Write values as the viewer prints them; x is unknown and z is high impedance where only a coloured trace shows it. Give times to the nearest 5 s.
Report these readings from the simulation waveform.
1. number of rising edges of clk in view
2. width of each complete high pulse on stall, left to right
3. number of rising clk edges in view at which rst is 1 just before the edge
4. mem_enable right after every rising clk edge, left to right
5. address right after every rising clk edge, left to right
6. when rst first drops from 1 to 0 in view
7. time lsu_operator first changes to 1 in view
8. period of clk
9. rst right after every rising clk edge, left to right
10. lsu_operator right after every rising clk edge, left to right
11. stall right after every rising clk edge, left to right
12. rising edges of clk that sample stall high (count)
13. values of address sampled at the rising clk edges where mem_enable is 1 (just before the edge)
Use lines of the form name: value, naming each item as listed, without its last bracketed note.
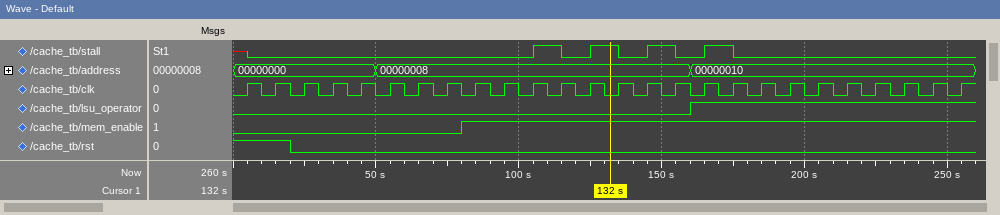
number of rising edges of clk in view: 26
width of each complete high pulse on stall, left to right: 10 s, 10 s, 10 s, 10 s
number of rising clk edges in view at which rst is 1 just before the edge: 2
mem_enable right after every rising clk edge, left to right: 0 0 0 0 0 0 0 0 1 1 1 1 1 1 1 1 1 1 1 1 1 1 1 1 1 1
address right after every rising clk edge, left to right: 00000000, 00000000, 00000000, 00000000, 00000000, 00000008, 00000008, 00000008, 00000008, 00000008, 00000008, 00000008, 00000008, 00000008, 00000008, 00000008, 00000010, 00000010, 00000010, 00000010, 00000010, 00000010, 00000010, 00000010, 00000010, 00000010
when rst first drops from 1 to 0 in view: 20 s
time lsu_operator first changes to 1 in view: 160 s
period of clk: 10 s
rst right after every rising clk edge, left to right: 1 1 0 0 0 0 0 0 0 0 0 0 0 0 0 0 0 0 0 0 0 0 0 0 0 0
lsu_operator right after every rising clk edge, left to right: 0 0 0 0 0 0 0 0 0 0 0 0 0 0 0 0 1 1 1 1 1 1 1 1 1 1
stall right after every rising clk edge, left to right: 0 0 0 0 0 0 0 0 0 0 1 0 1 0 1 0 1 0 0 0 0 0 0 0 0 0
rising edges of clk that sample stall high: 4
values of address sampled at the rising clk edges where mem_enable is 1: 00000008, 00000008, 00000008, 00000008, 00000008, 00000008, 00000008, 00000008, 00000010, 00000010, 00000010, 00000010, 00000010, 00000010, 00000010, 00000010, 00000010, 00000010
